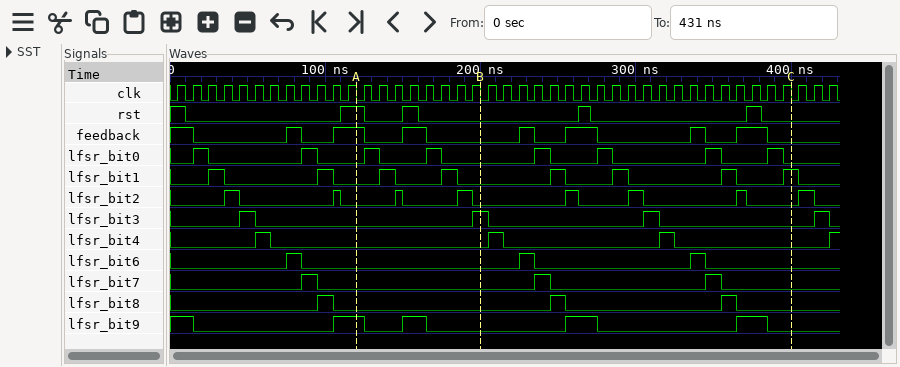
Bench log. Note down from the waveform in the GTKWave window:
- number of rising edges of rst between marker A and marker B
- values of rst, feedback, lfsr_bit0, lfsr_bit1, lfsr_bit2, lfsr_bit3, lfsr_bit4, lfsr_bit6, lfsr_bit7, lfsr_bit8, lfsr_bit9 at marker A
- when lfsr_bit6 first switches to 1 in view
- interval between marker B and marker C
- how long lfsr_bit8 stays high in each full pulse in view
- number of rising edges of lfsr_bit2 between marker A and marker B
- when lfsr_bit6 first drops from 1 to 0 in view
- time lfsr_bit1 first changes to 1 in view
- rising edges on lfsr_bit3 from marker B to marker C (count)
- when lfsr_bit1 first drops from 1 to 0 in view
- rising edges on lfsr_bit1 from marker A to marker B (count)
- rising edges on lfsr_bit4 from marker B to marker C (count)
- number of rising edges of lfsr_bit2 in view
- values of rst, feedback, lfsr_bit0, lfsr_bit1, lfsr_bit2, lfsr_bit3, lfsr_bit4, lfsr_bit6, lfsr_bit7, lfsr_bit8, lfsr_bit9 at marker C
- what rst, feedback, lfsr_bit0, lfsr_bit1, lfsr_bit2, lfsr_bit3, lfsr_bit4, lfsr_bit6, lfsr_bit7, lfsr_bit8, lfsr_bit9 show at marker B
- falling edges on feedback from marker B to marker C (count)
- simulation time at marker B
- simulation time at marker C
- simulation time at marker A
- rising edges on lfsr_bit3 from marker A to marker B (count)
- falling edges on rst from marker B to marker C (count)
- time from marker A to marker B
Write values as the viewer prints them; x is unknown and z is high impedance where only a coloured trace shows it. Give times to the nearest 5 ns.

1
rst=1, feedback=1, lfsr_bit0=0, lfsr_bit1=0, lfsr_bit2=0, lfsr_bit3=0, lfsr_bit4=0, lfsr_bit6=0, lfsr_bit7=0, lfsr_bit8=0, lfsr_bit9=1
75 ns
200 ns
10 ns, 10 ns, 10 ns
2
85 ns
25 ns
1
35 ns
2
2
8
rst=0, feedback=0, lfsr_bit0=0, lfsr_bit1=1, lfsr_bit2=0, lfsr_bit3=0, lfsr_bit4=0, lfsr_bit6=0, lfsr_bit7=0, lfsr_bit8=0, lfsr_bit9=0
rst=0, feedback=0, lfsr_bit0=0, lfsr_bit1=0, lfsr_bit2=0, lfsr_bit3=1, lfsr_bit4=0, lfsr_bit6=0, lfsr_bit7=0, lfsr_bit8=0, lfsr_bit9=0
4
200 ns
400 ns
120 ns
1
2
80 ns
